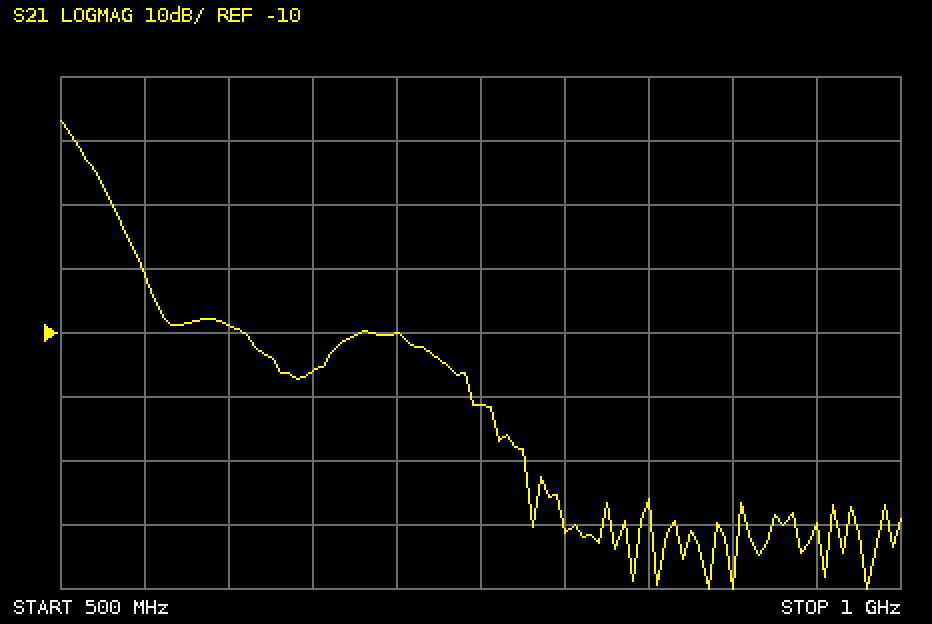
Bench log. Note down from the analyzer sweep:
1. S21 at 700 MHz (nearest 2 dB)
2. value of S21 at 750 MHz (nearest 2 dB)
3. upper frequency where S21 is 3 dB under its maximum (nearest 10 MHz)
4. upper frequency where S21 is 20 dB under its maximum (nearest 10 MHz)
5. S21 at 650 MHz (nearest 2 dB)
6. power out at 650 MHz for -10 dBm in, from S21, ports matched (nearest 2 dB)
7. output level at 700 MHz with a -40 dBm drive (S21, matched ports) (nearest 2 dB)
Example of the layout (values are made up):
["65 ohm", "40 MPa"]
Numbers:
["-10 dB", "-22 dB", "510 MHz", "540 MHz", "-16 dB", "-26 dBm", "-50 dBm"]
